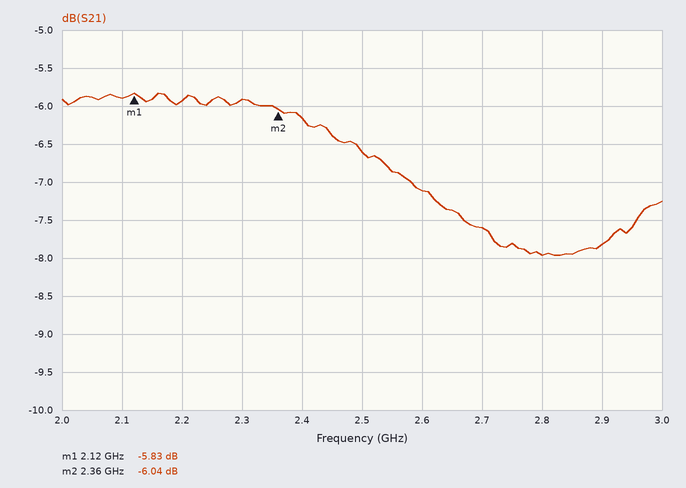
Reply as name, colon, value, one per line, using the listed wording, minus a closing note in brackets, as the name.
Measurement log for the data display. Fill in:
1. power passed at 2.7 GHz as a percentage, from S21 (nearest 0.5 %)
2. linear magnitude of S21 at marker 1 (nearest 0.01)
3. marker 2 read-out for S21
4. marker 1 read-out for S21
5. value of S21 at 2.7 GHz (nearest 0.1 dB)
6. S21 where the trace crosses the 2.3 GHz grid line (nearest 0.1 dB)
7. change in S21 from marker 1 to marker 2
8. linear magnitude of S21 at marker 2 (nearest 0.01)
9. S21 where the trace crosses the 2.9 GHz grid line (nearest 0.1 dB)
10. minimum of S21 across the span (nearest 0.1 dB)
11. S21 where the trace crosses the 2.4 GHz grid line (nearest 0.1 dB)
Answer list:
power passed at 2.7 GHz as a percentage, from S21: 17.5 %
linear magnitude of S21 at marker 1: 0.51
marker 2 read-out for S21: -6.04 dB
marker 1 read-out for S21: -5.83 dB
value of S21 at 2.7 GHz: -7.6 dB
S21 where the trace crosses the 2.3 GHz grid line: -5.9 dB
change in S21 from marker 1 to marker 2: -0.21 dB
linear magnitude of S21 at marker 2: 0.50
S21 where the trace crosses the 2.9 GHz grid line: -7.8 dB
minimum of S21 across the span: -8.0 dB
S21 where the trace crosses the 2.4 GHz grid line: -6.2 dB
